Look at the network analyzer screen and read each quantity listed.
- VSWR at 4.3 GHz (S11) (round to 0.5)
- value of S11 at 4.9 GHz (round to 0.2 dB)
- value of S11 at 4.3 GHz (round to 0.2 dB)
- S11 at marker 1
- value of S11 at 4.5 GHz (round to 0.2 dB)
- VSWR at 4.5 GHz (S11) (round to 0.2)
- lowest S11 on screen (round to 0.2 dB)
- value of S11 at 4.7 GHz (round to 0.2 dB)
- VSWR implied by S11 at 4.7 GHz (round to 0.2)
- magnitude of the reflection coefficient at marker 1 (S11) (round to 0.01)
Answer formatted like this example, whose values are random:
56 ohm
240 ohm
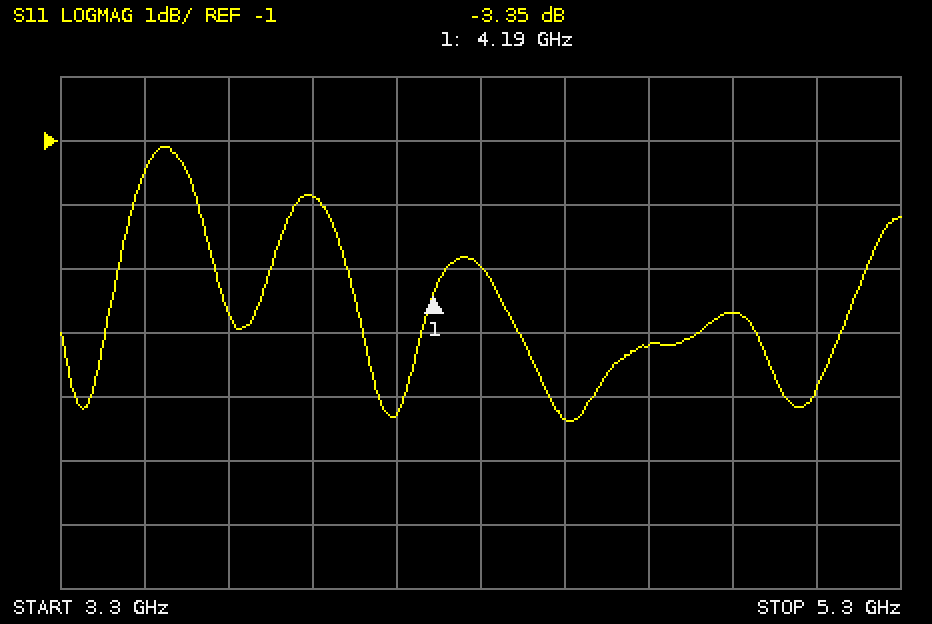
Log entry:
6.0
-3.6 dB
-3.0 dB
-3.35 dB
-5.4 dB
3.4
-5.4 dB
-4.2 dB
4.2
0.68
